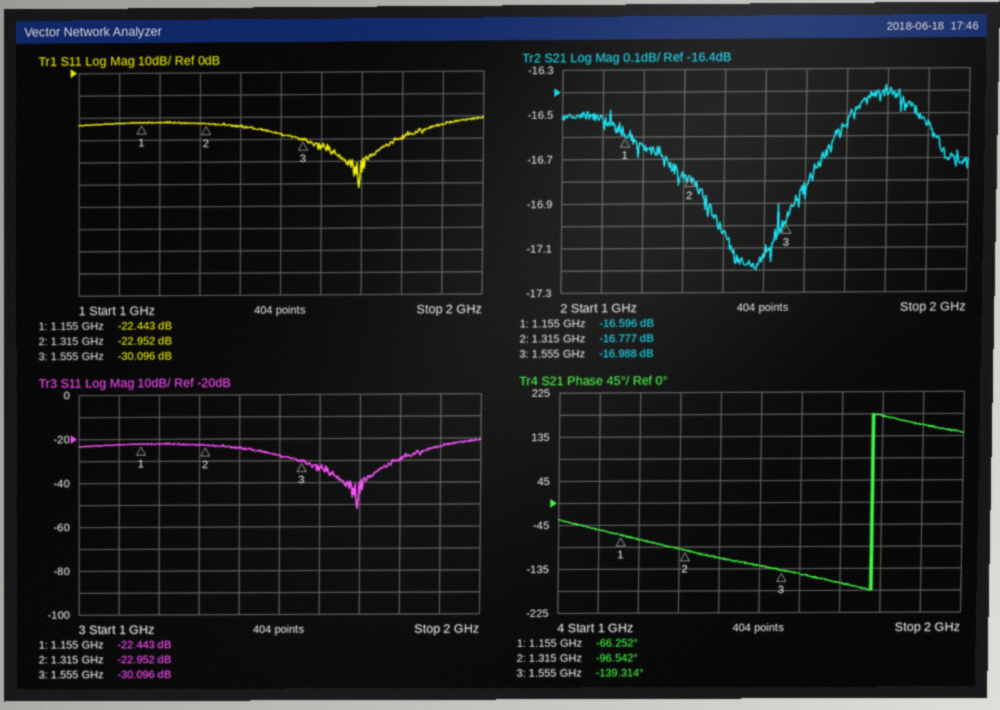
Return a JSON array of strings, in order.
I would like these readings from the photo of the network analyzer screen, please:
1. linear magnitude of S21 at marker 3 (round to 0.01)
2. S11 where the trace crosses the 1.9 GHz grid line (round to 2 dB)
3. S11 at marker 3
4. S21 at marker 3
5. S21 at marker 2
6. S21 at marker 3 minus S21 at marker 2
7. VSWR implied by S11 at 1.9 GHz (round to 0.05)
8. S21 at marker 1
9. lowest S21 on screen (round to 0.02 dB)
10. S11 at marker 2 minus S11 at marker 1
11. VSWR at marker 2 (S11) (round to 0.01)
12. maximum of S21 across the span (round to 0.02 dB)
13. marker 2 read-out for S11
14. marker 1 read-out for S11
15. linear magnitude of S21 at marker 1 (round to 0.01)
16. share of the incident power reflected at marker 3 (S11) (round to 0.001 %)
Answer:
["0.14", "-24 dB", "-30.096 dB", "-16.988 dB", "-16.777 dB", "-0.211 dB", "1.15", "-16.596 dB", "-17.20 dB", "-0.509 dB", "1.15", "-16.38 dB", "-22.952 dB", "-22.443 dB", "0.15", "0.098 %"]
